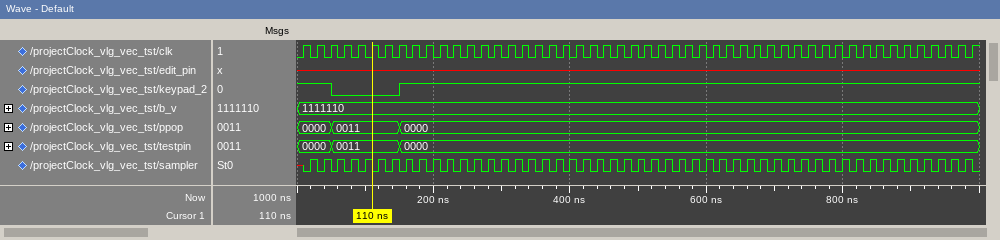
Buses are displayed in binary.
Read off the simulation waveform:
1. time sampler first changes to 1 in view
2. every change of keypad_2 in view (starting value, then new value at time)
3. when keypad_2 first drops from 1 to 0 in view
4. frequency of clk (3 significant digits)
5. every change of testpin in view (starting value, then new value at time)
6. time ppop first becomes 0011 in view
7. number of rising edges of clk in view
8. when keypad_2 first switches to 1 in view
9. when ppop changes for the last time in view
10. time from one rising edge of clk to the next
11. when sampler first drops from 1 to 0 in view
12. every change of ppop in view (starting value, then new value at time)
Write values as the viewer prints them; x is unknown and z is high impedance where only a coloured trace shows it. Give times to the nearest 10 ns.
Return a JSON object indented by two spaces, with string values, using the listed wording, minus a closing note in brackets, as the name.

{
  "time sampler first changes to 1 in view": "20 ns",
  "every change of keypad_2 in view": "1, 0 at 50 ns, 1 at 150 ns",
  "when keypad_2 first drops from 1 to 0 in view": "50 ns",
  "frequency of clk": "50.0 MHz",
  "every change of testpin in view": "0000, 0011 at 50 ns, 0000 at 150 ns",
  "time ppop first becomes 0011 in view": "50 ns",
  "number of rising edges of clk in view": "50",
  "when keypad_2 first switches to 1 in view": "150 ns",
  "when ppop changes for the last time in view": "150 ns",
  "time from one rising edge of clk to the next": "20 ns",
  "when sampler first drops from 1 to 0 in view": "30 ns",
  "every change of ppop in view": "0000, 0011 at 50 ns, 0000 at 150 ns"
}
